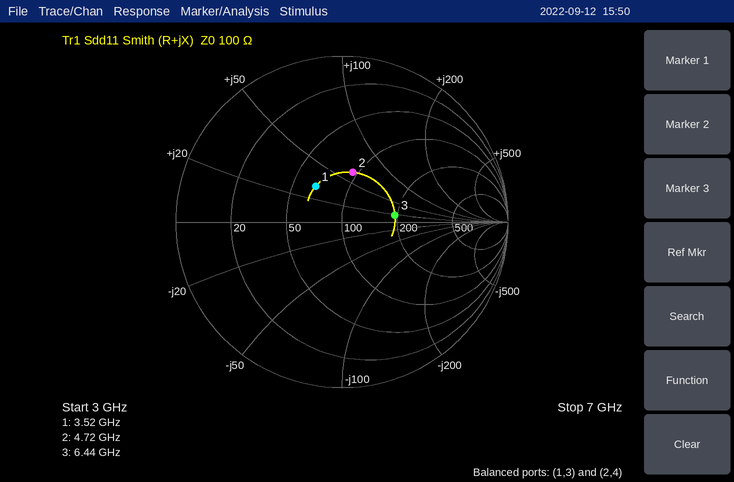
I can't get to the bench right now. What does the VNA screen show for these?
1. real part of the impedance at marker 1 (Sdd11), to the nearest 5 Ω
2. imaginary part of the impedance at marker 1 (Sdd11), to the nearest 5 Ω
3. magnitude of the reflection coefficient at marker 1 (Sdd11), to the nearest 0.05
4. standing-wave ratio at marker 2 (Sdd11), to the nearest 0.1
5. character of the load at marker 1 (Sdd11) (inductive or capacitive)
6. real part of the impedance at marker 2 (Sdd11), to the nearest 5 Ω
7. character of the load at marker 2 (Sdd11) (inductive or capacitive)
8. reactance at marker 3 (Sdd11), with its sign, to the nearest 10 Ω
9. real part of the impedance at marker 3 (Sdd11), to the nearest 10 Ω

65 Ω
+30 Ω
0.25
1.9
inductive
95 Ω
inductive
+20 Ω
190 Ω
